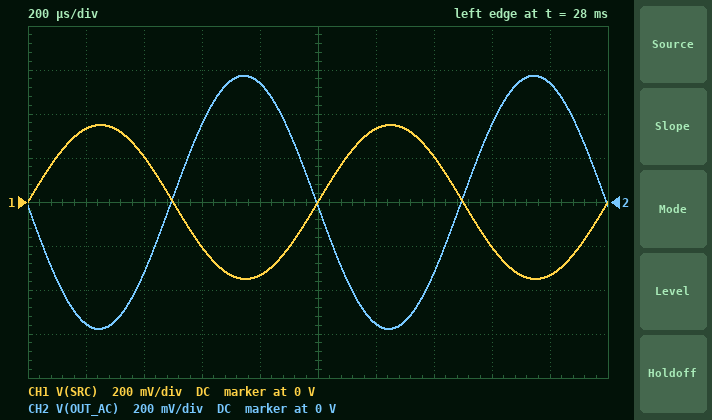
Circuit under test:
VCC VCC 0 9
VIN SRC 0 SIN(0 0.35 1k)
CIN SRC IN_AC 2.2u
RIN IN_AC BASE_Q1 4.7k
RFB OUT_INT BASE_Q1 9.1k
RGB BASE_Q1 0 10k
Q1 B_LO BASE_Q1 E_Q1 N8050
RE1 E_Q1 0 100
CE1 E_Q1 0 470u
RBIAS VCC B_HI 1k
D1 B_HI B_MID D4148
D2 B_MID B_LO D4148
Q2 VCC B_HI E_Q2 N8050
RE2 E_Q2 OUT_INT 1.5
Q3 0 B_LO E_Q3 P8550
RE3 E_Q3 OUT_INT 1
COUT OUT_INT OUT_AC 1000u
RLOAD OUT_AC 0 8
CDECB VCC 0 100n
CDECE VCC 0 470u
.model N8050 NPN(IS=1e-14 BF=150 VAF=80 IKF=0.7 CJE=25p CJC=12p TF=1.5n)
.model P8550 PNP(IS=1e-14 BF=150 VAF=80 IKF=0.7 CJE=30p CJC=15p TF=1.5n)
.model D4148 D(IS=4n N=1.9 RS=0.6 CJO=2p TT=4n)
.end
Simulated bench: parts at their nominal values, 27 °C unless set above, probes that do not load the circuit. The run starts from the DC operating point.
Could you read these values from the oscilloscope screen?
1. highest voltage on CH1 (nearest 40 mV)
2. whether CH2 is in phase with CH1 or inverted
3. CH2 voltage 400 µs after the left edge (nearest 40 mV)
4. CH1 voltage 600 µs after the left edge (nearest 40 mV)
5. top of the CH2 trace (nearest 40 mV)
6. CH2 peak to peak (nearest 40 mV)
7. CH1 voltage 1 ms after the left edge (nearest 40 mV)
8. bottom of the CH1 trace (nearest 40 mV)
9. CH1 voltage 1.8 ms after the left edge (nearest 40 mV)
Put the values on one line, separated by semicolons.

360 mV; inverted; -320 mV; -200 mV; 560 mV; 1.16 V; 0 V; -360 mV; -320 mV
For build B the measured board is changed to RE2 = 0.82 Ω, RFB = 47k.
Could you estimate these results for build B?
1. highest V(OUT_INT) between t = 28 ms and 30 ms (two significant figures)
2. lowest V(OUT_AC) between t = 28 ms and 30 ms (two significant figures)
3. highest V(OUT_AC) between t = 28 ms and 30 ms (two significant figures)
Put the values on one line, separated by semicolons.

7.0 V; -1.6 V; 1.1 V
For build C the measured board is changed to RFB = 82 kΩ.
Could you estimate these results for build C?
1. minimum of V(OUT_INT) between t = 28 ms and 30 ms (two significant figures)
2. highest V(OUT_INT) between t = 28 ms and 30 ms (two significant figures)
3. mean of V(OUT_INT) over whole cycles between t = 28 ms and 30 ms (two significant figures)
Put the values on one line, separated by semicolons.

5.6 V; 7.6 V; 7.0 V
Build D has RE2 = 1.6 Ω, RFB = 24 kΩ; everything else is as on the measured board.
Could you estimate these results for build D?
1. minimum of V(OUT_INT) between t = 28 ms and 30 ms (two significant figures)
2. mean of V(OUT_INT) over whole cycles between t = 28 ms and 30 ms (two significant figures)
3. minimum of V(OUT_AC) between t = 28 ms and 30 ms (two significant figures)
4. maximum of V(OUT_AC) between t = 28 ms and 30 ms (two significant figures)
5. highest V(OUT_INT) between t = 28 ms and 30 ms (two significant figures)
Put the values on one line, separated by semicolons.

3.1 V; 4.3 V; -1.2 V; 1.2 V; 5.5 V
